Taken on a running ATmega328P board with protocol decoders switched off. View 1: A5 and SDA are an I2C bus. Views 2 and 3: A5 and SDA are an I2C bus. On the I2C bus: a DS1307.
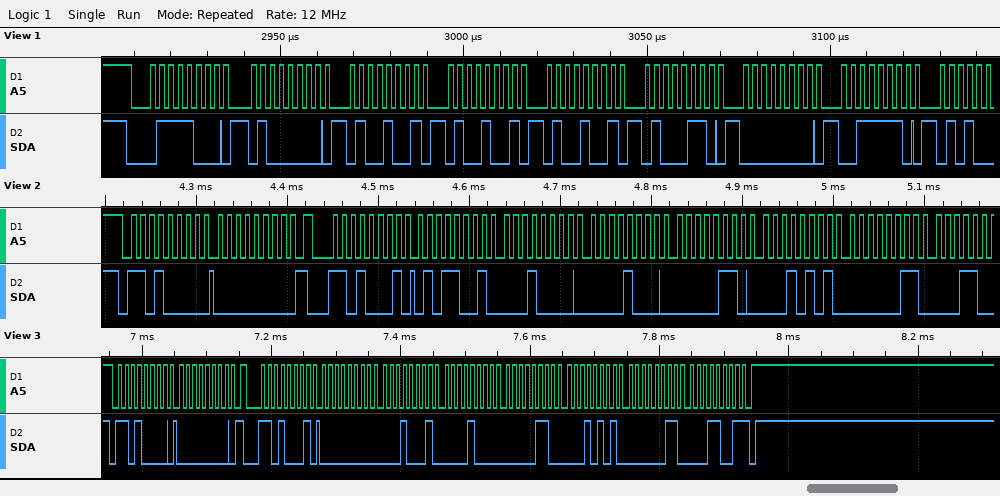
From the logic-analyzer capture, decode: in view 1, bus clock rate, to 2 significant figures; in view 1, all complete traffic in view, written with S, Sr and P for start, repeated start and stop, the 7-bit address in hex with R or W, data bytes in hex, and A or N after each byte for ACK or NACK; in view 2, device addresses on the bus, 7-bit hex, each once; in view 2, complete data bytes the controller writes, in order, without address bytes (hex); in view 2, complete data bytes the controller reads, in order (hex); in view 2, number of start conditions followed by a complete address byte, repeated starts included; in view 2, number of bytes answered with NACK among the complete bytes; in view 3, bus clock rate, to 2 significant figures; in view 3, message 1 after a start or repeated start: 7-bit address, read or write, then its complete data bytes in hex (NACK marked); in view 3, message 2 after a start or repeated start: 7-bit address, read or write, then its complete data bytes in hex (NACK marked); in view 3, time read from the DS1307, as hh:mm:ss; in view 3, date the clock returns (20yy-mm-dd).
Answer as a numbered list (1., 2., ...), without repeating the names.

1. 400 kHz
2. S 3CW A 40 A 49 A 49 A 49 A 46 A 00 A 3E A
3. 0x68
4. 00
5. 59 10 08 06 15 03
6. 2
7. 0
8. 100 kHz
9. 0x68 write: 00
10. 0x68 read: 00 11 08 06 15 03 19 NACK
11. 08:11:00
12. 2019-03-15
